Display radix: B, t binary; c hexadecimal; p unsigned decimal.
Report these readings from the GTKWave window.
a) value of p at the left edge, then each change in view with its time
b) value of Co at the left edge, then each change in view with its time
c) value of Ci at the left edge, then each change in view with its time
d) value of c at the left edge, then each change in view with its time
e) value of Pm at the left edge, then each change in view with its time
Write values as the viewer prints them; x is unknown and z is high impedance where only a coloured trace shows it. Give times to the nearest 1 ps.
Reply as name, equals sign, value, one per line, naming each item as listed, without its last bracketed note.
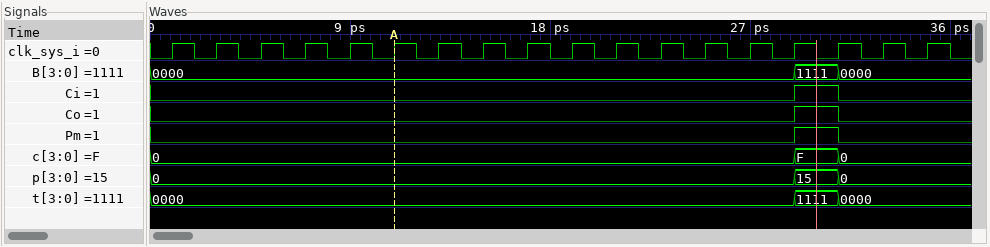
value of p at the left edge, then each change in view with its time = 0, 15 at 29 ps, 0 at 31 ps
value of Co at the left edge, then each change in view with its time = 0, 1 at 29 ps, 0 at 31 ps
value of Ci at the left edge, then each change in view with its time = 0, 1 at 29 ps, 0 at 31 ps
value of c at the left edge, then each change in view with its time = 0, F at 29 ps, 0 at 31 ps
value of Pm at the left edge, then each change in view with its time = 0, 1 at 29 ps, 0 at 31 ps
